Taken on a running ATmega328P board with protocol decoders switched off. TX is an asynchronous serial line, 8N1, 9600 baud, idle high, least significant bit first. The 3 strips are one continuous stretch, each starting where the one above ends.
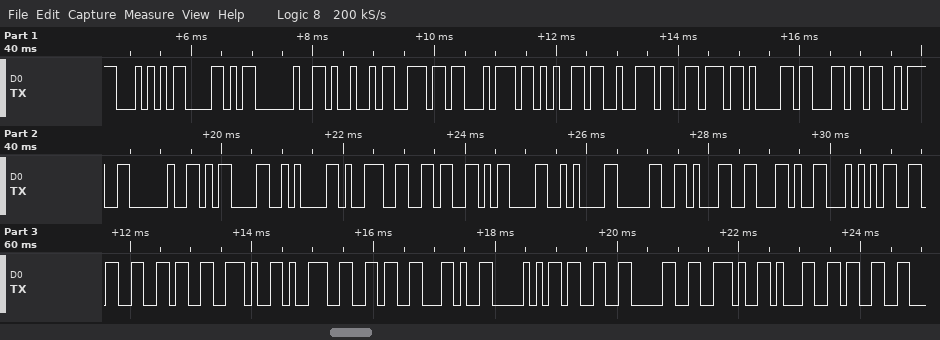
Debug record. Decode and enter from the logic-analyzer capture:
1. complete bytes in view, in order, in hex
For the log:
54 58 20 49 6E 74 65 72 76 61 6C 3A 20 0D 0A 39 36 0D 0A 30 31 2C 54 36 36 2E 39 36 2C 50 33 30 2E 31 33
